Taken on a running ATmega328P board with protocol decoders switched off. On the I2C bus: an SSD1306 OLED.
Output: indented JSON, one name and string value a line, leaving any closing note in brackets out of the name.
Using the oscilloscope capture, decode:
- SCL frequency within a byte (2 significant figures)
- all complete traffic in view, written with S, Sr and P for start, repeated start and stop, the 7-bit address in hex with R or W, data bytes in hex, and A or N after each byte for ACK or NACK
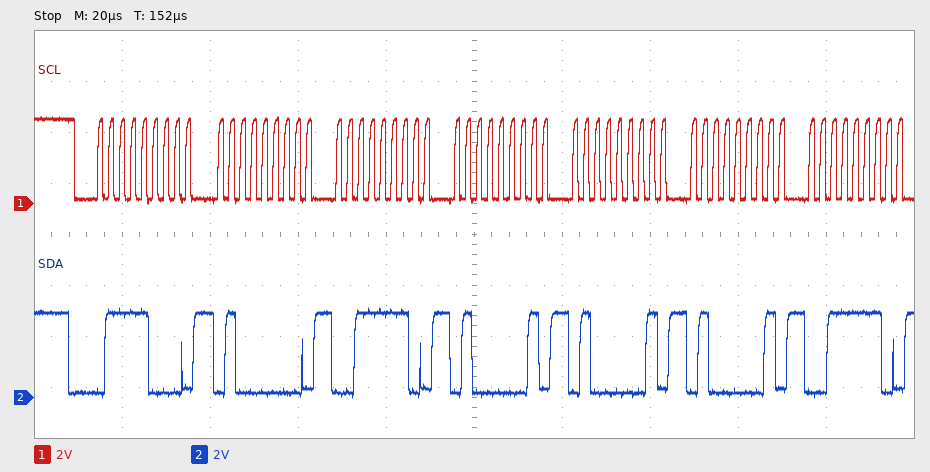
{
  "SCL frequency within a byte": "400 kHz",
  "all complete traffic in view, written with S, Sr and P for start, repeated start and stop, the 7-bit address in hex with R or W, data bytes in hex, and A or N after each byte for ACK or NACK": "S 3CW A 40 A 3E A 41 A 41 A 41 A 3E A"
}
